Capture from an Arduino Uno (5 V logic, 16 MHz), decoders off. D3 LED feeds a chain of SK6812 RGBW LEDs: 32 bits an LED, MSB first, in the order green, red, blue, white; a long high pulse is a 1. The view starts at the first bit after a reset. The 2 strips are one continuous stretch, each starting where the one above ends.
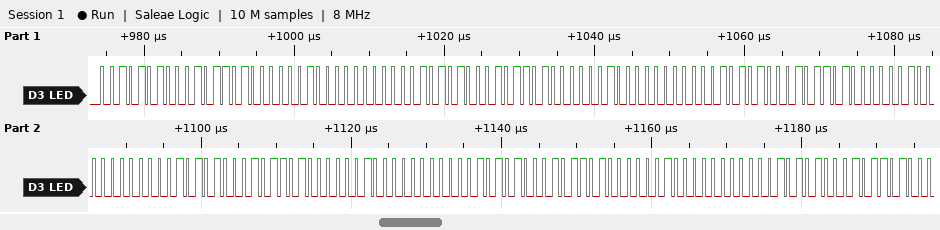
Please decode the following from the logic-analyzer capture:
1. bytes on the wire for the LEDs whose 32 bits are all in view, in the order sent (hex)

2A 2D 02 00 2A 2D 02 00 2A 2D 02 00 2A 2D 02 00 2A 2D 02 00
